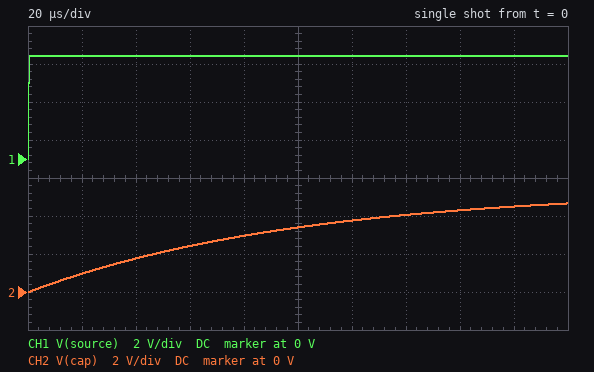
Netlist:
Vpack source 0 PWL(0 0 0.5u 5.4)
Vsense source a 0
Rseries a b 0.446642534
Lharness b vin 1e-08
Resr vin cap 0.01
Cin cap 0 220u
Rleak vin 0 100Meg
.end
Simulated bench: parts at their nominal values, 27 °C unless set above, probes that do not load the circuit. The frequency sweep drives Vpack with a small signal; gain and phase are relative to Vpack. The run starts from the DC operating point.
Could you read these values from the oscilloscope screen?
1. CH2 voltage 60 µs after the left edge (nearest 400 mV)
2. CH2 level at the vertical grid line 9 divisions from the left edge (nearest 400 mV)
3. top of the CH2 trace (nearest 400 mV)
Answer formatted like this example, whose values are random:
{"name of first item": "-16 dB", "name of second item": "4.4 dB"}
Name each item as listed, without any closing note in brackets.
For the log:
{"CH2 voltage 60 µs after the left edge": "2.4 V", "CH2 level at the vertical grid line 9 divisions from the left edge": "4.4 V", "top of the CH2 trace": "4.8 V"}
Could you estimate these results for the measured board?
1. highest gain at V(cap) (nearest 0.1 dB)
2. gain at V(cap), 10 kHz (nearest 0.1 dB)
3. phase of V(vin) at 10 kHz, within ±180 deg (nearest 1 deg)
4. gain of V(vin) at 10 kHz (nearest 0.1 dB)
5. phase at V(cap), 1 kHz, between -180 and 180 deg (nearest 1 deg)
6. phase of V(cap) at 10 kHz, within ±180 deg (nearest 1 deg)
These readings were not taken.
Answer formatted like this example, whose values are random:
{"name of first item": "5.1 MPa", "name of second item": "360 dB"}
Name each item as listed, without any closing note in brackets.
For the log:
{"highest gain at V(cap)": "0 dB", "gain at V(cap), 10 kHz": "-16.1 dB", "phase of V(vin) at 10 kHz, within ±180 deg": "-73 deg", "gain of V(vin) at 10 kHz": "-16.0 dB", "phase at V(cap), 1 kHz, between -180 and 180 deg": "-32 deg", "phase of V(cap) at 10 kHz, within ±180 deg": "-81 deg"}
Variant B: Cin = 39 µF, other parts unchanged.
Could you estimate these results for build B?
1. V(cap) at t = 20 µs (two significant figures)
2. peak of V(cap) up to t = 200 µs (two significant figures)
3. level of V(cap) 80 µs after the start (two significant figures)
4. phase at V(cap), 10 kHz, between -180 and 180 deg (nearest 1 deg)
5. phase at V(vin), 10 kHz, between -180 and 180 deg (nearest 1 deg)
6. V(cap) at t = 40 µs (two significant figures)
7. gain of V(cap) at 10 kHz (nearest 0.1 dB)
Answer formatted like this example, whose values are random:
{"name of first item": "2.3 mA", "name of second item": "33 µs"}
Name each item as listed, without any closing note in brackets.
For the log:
{"V(cap) at t = 20 µs": "3.6 V", "peak of V(cap) up to t = 200 µs": "5.4 V", "level of V(cap) 80 µs after the start": "5.3 V", "phase at V(cap), 10 kHz, between -180 and 180 deg": "-48 deg", "phase at V(vin), 10 kHz, between -180 and 180 deg": "-47 deg", "V(cap) at t = 40 µs": "4.8 V", "gain of V(cap) at 10 kHz": "-3.5 dB"}
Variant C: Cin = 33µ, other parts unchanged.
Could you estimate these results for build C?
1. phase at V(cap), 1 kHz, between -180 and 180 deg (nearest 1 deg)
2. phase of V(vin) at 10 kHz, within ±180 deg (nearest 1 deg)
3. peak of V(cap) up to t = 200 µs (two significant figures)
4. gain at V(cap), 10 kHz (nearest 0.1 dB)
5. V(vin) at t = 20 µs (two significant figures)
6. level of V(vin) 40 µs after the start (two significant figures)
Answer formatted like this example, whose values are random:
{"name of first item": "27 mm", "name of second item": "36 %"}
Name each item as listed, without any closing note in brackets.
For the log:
{"phase at V(cap), 1 kHz, between -180 and 180 deg": "-5 deg", "phase of V(vin) at 10 kHz, within ±180 deg": "-42 deg", "peak of V(cap) up to t = 200 µs": "5.4 V", "gain at V(cap), 10 kHz": "-2.8 dB", "V(vin) at t = 20 µs": "4.0 V", "level of V(vin) 40 µs after the start": "5.0 V"}
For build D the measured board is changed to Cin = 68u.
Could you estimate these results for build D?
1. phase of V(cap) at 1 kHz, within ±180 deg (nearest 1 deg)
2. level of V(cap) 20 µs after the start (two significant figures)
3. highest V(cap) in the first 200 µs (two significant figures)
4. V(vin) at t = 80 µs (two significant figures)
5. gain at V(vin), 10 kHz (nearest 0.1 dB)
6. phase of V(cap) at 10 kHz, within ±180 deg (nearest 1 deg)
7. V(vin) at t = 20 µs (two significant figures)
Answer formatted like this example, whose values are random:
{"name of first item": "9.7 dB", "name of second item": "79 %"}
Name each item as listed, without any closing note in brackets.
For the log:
{"phase of V(cap) at 1 kHz, within ±180 deg": "-11 deg", "level of V(cap) 20 µs after the start": "2.5 V", "highest V(cap) in the first 200 µs": "5.4 V", "V(vin) at t = 80 µs": "5.0 V", "gain at V(vin), 10 kHz": "-6.8 dB", "phase of V(cap) at 10 kHz, within ±180 deg": "-63 deg", "V(vin) at t = 20 µs": "2.6 V"}
